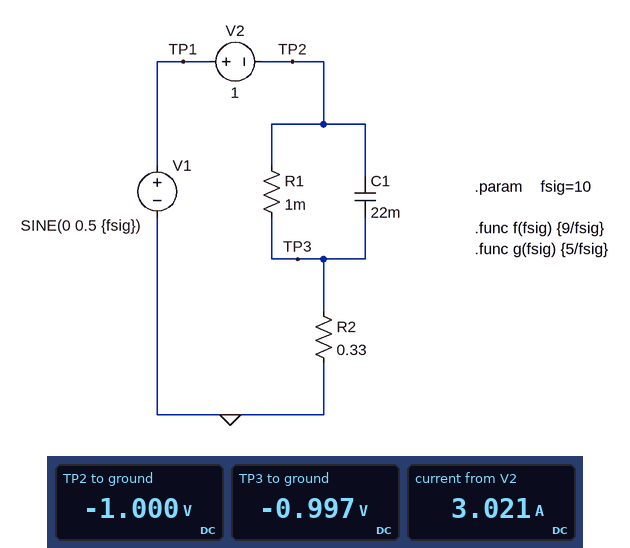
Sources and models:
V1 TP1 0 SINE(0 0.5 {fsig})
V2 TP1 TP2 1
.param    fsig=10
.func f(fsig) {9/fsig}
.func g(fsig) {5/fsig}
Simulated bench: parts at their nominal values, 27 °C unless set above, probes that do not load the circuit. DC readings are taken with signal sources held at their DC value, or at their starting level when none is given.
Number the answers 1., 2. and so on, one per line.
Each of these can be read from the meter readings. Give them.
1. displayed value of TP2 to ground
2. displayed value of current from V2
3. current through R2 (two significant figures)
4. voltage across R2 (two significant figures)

1. -1.000 V
2. 3.021 A
3. 3.0 A
4. 1.0 V
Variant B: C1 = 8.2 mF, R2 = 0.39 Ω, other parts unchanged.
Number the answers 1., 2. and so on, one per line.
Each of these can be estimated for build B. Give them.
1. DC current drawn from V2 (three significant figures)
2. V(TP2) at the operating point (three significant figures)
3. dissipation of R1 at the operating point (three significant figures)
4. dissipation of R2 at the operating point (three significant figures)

1. 2.56 A
2. -1.00 V
3. 6.54 mW
4. 2.55 W
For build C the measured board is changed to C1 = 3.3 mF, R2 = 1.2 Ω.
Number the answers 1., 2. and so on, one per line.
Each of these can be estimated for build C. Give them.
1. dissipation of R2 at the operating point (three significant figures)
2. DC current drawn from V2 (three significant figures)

1. 832 mW
2. 833 mA
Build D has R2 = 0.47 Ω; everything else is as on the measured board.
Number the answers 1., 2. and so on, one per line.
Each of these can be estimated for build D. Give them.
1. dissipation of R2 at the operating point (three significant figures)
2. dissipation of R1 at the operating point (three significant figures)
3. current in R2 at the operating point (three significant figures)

1. 2.12 W
2. 4.51 mW
3. 2.12 A
